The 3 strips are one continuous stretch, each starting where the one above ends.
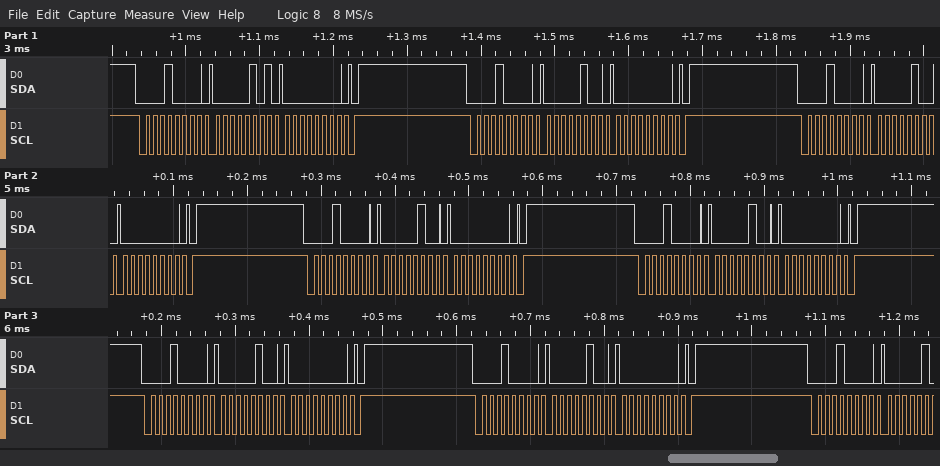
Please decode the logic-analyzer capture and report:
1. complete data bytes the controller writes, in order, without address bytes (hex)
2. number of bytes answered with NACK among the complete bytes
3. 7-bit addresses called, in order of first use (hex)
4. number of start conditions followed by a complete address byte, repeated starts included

05 00 04 00 04 00 04 00 04 00 04 00 04 00
0
0x08
8
